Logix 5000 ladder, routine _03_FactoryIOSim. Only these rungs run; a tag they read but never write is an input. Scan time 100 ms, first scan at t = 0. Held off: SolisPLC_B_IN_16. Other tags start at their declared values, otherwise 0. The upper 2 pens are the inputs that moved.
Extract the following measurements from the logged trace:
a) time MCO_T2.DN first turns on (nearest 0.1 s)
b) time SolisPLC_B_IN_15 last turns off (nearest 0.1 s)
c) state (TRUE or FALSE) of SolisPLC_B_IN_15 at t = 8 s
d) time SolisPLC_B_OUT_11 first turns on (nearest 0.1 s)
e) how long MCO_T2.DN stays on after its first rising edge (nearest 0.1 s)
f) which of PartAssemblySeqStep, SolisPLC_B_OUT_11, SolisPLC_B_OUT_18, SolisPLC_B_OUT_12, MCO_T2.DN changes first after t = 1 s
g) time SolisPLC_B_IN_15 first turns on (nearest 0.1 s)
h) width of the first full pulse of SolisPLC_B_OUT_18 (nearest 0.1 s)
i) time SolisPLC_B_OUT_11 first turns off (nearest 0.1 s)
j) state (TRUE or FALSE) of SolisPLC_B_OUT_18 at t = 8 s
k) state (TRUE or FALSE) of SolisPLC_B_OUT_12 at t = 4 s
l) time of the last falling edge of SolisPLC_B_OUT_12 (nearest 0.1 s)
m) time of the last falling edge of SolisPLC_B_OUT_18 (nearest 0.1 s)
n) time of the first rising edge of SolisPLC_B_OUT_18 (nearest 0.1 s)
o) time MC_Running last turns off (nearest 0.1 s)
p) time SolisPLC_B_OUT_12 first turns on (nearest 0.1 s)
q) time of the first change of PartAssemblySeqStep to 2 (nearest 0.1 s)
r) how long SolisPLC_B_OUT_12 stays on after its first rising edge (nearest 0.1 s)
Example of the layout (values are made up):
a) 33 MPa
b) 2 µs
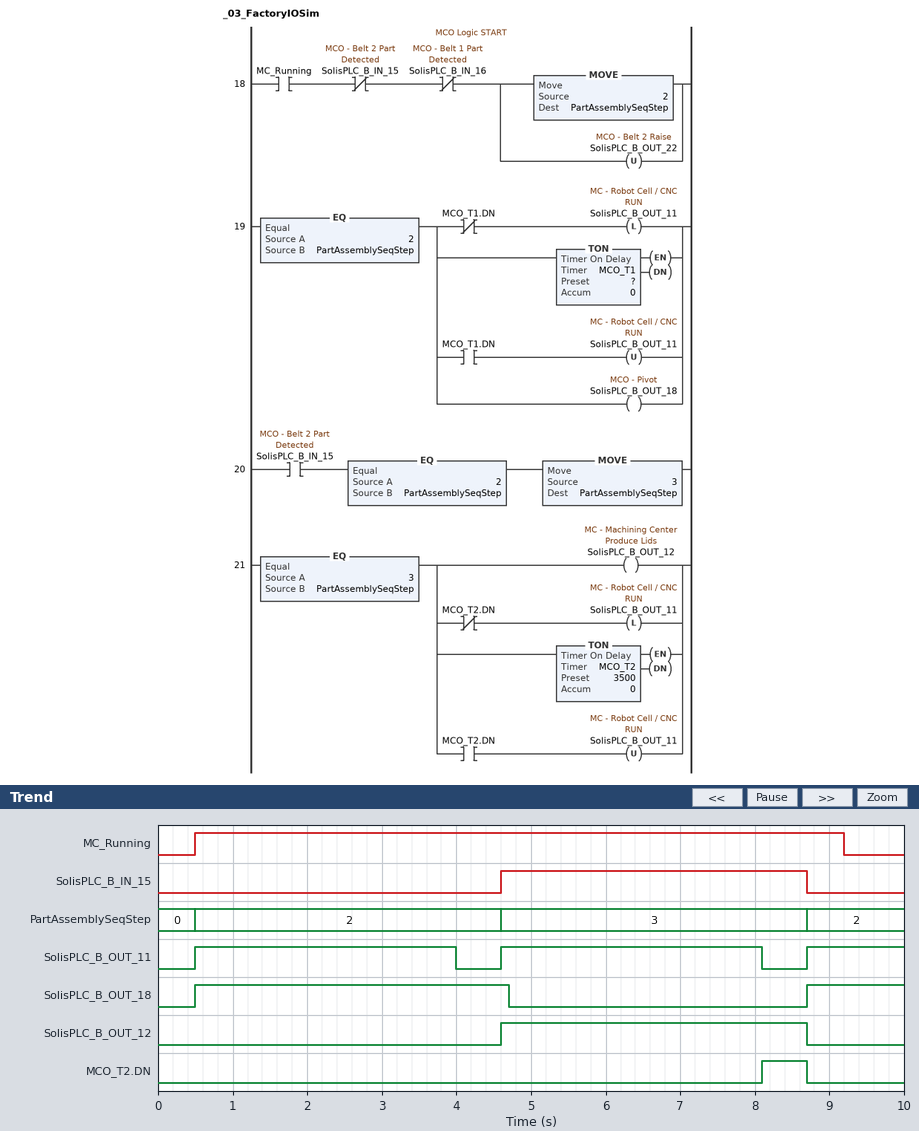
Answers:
a) 8.1 s
b) 8.7 s
c) TRUE
d) 0.5 s
e) 0.6 s
f) SolisPLC_B_OUT_11
g) 4.6 s
h) 4.2 s
i) 4.0 s
j) FALSE
k) FALSE
l) 8.7 s
m) 4.7 s
n) 0.5 s
o) 9.2 s
p) 4.6 s
q) 0.5 s
r) 4.1 s
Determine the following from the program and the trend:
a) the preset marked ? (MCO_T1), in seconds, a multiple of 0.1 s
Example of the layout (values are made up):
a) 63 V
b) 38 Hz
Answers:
a) 3.5 s
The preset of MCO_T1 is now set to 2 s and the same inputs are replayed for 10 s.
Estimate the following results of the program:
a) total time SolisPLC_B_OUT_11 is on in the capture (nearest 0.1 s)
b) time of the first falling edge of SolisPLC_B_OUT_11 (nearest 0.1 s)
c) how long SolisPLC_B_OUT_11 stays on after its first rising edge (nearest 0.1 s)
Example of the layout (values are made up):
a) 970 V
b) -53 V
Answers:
a) 6.8 s
b) 2.5 s
c) 2.0 s
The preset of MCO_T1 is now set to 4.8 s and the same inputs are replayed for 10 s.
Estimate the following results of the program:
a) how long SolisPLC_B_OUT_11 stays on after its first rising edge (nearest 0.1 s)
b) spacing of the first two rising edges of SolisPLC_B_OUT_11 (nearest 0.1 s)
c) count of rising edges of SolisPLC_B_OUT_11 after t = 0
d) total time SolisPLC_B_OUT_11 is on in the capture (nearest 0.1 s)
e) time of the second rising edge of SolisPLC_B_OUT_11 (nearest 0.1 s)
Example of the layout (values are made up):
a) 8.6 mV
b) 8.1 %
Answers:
a) 7.6 s
b) 8.2 s
c) 2
d) 8.9 s
e) 8.7 s
